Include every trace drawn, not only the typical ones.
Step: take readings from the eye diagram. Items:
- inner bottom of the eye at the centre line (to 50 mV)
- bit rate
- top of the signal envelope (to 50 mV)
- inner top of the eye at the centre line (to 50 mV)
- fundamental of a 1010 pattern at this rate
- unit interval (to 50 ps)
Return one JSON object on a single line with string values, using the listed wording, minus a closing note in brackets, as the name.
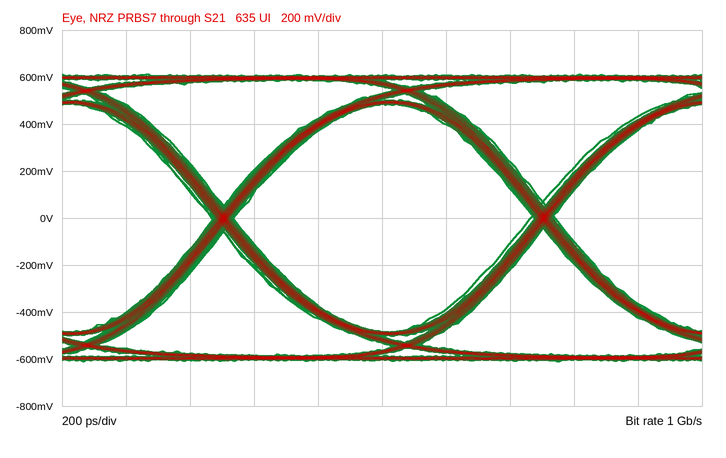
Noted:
{"inner bottom of the eye at the centre line": "-500 mV", "bit rate": "1 Gb/s", "top of the signal envelope": "600 mV", "inner top of the eye at the centre line": "500 mV", "fundamental of a 1010 pattern at this rate": "500 MHz", "unit interval": "1.00 ns"}
